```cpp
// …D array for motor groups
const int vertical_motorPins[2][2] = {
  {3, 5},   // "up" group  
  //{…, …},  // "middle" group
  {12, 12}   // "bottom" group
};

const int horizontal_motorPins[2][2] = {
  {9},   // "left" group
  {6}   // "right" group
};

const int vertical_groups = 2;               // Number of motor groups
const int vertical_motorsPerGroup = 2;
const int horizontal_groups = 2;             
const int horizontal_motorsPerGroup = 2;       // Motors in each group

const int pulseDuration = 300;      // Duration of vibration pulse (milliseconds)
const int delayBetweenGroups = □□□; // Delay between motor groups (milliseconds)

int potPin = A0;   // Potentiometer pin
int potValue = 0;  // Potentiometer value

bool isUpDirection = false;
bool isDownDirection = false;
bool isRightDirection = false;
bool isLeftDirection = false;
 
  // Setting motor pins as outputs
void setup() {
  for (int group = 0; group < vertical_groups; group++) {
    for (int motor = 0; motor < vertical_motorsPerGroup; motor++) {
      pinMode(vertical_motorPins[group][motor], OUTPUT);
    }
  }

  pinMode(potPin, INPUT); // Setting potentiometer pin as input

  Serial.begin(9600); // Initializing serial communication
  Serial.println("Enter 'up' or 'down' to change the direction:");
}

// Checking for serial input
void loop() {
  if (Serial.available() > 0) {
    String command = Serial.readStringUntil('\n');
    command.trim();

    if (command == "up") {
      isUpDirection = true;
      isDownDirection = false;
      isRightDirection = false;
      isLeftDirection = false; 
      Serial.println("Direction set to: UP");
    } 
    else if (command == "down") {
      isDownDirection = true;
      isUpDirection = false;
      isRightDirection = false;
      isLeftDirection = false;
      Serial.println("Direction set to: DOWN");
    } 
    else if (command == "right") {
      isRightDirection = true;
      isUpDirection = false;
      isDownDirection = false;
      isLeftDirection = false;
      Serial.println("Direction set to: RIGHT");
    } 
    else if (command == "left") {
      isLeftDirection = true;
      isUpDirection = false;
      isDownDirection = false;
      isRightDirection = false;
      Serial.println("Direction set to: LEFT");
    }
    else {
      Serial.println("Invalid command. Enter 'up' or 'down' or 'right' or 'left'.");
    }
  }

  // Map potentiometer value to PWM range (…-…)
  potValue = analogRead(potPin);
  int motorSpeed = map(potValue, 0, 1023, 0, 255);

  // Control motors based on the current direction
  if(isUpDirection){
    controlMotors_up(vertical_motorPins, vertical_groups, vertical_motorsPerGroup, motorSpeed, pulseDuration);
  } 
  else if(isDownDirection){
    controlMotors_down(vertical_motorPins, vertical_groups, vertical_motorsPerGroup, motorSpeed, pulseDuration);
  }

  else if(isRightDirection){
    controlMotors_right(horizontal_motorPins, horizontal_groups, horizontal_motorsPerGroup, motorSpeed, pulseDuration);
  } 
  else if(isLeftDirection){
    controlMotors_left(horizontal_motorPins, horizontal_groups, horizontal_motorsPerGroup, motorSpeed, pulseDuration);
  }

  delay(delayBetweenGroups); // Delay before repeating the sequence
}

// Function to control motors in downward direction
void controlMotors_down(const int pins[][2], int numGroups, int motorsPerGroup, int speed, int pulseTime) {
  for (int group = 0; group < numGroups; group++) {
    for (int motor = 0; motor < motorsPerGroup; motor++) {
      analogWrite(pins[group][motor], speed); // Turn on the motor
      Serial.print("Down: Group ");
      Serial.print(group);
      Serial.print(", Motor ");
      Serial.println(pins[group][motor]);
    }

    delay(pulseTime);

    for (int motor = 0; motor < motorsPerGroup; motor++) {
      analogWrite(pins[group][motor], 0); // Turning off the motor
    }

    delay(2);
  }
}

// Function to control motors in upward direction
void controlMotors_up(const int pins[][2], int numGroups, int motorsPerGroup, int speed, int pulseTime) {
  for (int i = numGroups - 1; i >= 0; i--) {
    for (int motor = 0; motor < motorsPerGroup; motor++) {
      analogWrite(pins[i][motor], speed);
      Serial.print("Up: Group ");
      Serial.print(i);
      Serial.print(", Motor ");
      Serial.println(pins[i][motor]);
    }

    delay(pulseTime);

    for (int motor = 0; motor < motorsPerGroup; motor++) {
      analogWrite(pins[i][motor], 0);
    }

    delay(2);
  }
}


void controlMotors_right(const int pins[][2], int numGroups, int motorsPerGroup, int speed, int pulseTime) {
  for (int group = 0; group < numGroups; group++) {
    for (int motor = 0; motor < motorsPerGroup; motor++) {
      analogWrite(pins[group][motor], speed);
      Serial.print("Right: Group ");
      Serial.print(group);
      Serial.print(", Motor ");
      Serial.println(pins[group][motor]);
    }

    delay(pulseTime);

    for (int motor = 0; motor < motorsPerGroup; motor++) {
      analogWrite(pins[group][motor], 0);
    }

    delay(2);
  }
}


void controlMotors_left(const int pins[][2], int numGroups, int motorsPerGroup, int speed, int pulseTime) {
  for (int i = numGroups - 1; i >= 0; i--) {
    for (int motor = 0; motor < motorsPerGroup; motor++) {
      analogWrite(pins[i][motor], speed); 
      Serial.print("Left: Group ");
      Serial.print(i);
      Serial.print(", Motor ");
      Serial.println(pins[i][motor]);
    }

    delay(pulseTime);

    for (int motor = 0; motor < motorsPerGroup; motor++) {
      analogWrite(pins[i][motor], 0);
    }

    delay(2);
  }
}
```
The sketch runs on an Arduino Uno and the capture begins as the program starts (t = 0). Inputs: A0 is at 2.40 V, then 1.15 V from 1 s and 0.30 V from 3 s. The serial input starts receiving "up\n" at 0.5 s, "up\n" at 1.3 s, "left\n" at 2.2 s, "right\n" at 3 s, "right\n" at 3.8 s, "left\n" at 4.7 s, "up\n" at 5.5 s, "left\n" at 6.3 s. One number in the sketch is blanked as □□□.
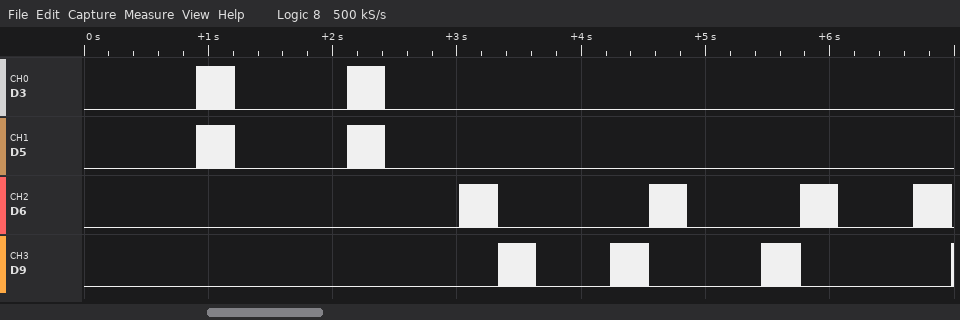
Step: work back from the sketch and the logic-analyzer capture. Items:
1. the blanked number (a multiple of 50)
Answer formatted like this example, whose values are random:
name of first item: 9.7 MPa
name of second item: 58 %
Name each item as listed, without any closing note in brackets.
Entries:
the blanked number: 600
